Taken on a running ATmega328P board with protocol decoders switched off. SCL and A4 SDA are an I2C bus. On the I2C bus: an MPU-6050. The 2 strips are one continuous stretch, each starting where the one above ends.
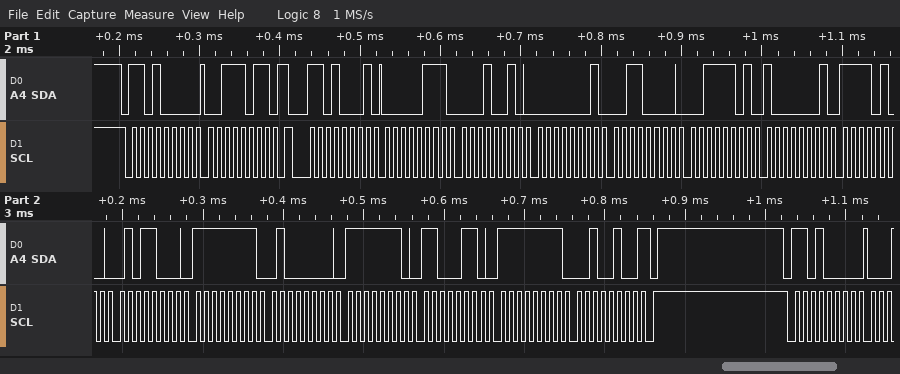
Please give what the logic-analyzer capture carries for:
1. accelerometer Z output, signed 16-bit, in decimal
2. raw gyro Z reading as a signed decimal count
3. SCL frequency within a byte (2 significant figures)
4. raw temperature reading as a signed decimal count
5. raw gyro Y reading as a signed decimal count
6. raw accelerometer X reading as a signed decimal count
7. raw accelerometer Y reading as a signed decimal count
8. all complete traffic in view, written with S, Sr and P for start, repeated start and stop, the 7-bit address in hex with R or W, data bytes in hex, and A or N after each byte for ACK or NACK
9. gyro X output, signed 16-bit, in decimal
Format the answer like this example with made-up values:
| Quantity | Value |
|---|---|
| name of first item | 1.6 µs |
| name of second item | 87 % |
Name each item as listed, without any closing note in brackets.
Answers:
| Quantity | Value |
|---|---|
| accelerometer Z output, signed 16-bit, in decimal | 15745 |
| raw gyro Z reading as a signed decimal count | -220 |
| SCL frequency within a byte | 100 kHz |
| raw temperature reading as a signed decimal count | -2984 |
| raw gyro Y reading as a signed decimal count | -314 |
| raw accelerometer X reading as a signed decimal count | 1810 |
| raw accelerometer Y reading as a signed decimal count | 304 |
| all complete traffic in view, written with S, Sr and P for start, repeated start and stop, the 7-bit address in hex with R or W, data bytes in hex, and A or N after each byte for ACK or NACK | S 68W A 3B A Sr 68R A 07 A 12 A 01 A 30 A 3D A 81 A F4 A 58 A FF A 40 A FE A C6 A FF A 24 N P S 68W A |
| gyro X output, signed 16-bit, in decimal | -192 |
